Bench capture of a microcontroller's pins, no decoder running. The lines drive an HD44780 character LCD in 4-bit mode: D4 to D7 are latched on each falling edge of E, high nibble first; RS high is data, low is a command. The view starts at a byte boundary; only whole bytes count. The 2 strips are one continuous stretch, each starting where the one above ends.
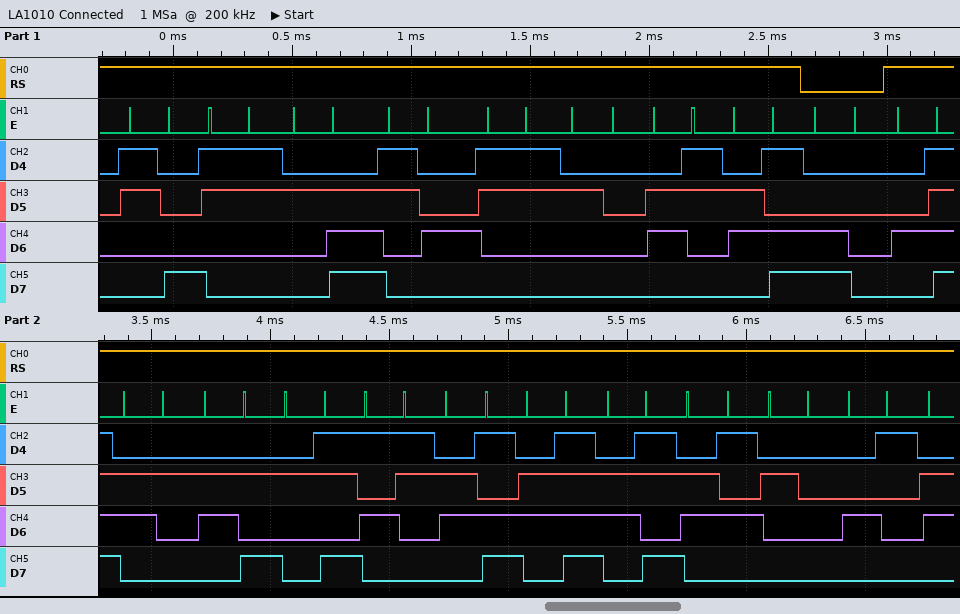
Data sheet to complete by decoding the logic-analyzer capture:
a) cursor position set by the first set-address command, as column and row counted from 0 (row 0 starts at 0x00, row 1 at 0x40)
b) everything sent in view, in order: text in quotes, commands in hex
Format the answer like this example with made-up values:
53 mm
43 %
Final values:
column 0, row 1
"83.43 cm" 0xC0 "Obj+Smoke A"
